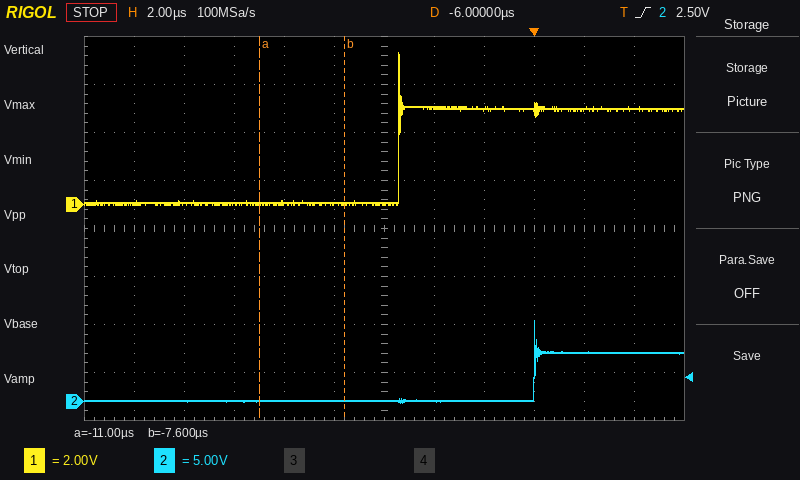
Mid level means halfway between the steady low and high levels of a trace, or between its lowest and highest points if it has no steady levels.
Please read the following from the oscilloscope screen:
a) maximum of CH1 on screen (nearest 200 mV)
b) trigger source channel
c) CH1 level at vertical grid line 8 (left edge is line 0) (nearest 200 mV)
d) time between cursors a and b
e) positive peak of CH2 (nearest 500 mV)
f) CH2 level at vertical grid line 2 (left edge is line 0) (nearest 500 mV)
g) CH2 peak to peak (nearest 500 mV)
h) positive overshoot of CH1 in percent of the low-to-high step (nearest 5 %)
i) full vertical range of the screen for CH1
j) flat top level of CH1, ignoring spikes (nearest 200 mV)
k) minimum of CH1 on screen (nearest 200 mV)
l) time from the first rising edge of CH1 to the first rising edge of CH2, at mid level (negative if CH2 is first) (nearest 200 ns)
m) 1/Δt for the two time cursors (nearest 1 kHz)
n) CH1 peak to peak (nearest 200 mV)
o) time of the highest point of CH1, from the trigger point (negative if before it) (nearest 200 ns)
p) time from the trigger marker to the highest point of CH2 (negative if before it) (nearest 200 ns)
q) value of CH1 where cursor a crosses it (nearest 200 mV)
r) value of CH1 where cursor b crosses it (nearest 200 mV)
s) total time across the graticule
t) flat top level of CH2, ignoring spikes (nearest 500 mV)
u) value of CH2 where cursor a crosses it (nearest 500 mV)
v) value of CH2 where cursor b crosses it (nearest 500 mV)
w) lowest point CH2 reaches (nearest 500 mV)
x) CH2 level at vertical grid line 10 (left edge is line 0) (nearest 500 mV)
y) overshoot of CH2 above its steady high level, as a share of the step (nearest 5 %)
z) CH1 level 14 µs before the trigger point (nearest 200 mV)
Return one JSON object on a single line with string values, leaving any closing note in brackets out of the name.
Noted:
{"maximum of CH1 on screen": "6.4 V", "trigger source channel": "CH2", "CH1 level at vertical grid line 8 (left edge is line 0)": "4.0 V", "time between cursors a and b": "3.4 µs", "positive peak of CH2": "8.5 V", "CH2 level at vertical grid line 2 (left edge is line 0)": "0.0 V", "CH2 peak to peak": "8.5 V", "positive overshoot of CH1 in percent of the low-to-high step": "60 %", "full vertical range of the screen for CH1": "16 V", "flat top level of CH1, ignoring spikes": "4.0 V", "minimum of CH1 on screen": "0.0 V", "time from the first rising edge of CH1 to the first rising edge of CH2, at mid level (negative if CH2 is first)": "+5.4 µs", "1/Δt for the two time cursors": "294 kHz", "CH1 peak to peak": "6.4 V", "time of the highest point of CH1, from the trigger point (negative if before it)": "-5.4 µs", "time from the trigger marker to the highest point of CH2 (negative if before it)": "0.0 µs", "value of CH1 where cursor a crosses it": "0.0 V", "value of CH1 where cursor b crosses it": "0.0 V", "total time across the graticule": "24 µs", "flat top level of CH2, ignoring spikes": "5.0 V", "value of CH2 where cursor a crosses it": "0.0 V", "value of CH2 where cursor b crosses it": "0.0 V", "lowest point CH2 reaches": "0.0 V", "CH2 level at vertical grid line 10 (left edge is line 0)": "5.0 V", "overshoot of CH2 above its steady high level, as a share of the step": "65 %", "CH1 level 14 µs before the trigger point": "0.0 V"}
